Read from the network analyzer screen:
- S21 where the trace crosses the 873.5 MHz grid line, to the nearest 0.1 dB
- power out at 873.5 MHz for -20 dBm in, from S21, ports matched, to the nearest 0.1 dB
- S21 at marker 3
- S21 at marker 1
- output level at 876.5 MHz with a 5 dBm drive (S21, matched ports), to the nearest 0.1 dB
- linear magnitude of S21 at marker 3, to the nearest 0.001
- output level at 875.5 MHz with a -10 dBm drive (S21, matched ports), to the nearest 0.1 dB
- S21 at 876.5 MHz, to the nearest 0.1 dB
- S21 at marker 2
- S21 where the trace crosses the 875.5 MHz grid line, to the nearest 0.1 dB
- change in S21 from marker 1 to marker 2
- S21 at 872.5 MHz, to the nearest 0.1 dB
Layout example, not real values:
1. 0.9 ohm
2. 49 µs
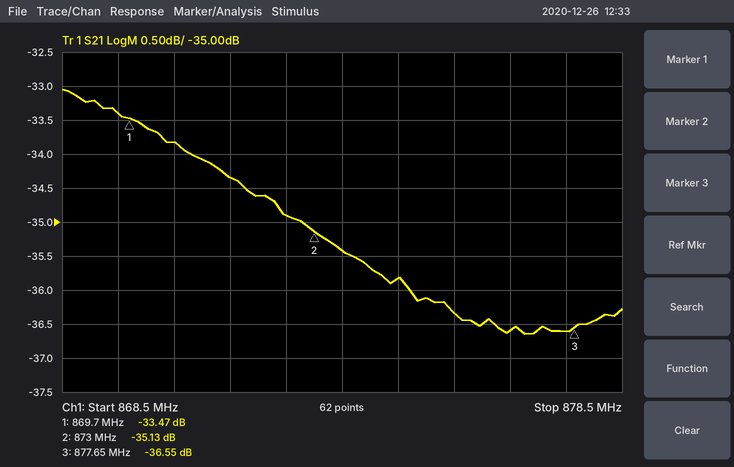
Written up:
1. -35.4 dB
2. -55.4 dBm
3. -36.55 dB
4. -33.47 dB
5. -31.6 dBm
6. 0.015
7. -46.3 dBm
8. -36.6 dB
9. -35.13 dB
10. -36.3 dB
11. -1.66 dB
12. -34.9 dB
